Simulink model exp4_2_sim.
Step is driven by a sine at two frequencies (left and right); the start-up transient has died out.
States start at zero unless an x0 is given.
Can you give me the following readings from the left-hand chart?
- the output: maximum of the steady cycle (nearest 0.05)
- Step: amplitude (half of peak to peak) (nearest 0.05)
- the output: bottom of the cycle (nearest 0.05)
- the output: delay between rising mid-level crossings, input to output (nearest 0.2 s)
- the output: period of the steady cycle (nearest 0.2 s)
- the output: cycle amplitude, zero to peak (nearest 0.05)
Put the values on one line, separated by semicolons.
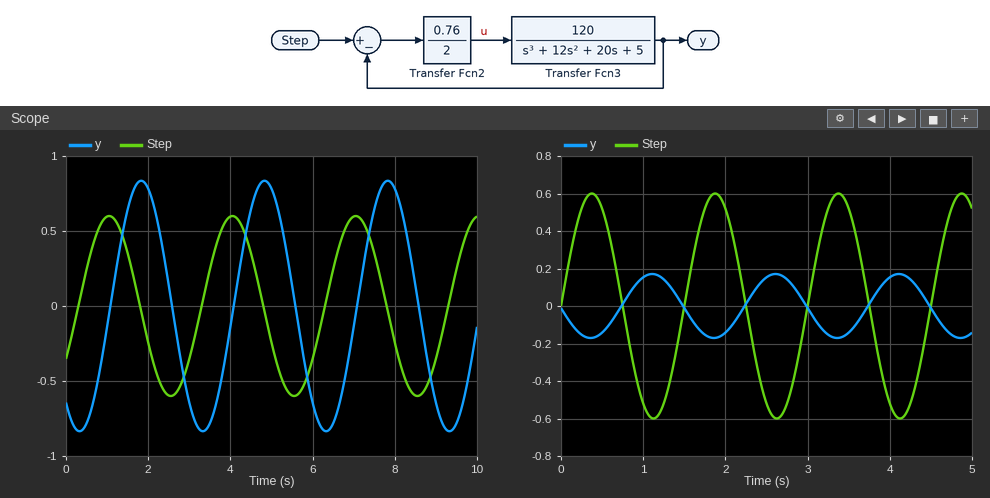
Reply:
0.85; 0.60; -0.85; 0.8 s; 3.0 s; 0.85
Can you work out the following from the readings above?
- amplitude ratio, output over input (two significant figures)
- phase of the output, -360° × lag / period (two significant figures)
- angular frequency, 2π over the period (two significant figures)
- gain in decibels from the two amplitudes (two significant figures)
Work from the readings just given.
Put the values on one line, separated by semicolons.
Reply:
1.4; -96°; 2.1 rad/s; 3.0 dB
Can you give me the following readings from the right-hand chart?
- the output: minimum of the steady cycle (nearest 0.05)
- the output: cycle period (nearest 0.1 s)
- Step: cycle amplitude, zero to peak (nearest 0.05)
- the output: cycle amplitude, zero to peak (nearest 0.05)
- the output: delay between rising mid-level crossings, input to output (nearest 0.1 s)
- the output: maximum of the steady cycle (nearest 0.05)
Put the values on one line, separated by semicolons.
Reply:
-0.15; 1.5 s; 0.60; 0.15; 0.7 s; 0.15
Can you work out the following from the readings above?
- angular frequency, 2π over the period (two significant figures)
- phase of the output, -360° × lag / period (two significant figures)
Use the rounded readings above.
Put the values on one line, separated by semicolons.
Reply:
4.2 rad/s; -170°
